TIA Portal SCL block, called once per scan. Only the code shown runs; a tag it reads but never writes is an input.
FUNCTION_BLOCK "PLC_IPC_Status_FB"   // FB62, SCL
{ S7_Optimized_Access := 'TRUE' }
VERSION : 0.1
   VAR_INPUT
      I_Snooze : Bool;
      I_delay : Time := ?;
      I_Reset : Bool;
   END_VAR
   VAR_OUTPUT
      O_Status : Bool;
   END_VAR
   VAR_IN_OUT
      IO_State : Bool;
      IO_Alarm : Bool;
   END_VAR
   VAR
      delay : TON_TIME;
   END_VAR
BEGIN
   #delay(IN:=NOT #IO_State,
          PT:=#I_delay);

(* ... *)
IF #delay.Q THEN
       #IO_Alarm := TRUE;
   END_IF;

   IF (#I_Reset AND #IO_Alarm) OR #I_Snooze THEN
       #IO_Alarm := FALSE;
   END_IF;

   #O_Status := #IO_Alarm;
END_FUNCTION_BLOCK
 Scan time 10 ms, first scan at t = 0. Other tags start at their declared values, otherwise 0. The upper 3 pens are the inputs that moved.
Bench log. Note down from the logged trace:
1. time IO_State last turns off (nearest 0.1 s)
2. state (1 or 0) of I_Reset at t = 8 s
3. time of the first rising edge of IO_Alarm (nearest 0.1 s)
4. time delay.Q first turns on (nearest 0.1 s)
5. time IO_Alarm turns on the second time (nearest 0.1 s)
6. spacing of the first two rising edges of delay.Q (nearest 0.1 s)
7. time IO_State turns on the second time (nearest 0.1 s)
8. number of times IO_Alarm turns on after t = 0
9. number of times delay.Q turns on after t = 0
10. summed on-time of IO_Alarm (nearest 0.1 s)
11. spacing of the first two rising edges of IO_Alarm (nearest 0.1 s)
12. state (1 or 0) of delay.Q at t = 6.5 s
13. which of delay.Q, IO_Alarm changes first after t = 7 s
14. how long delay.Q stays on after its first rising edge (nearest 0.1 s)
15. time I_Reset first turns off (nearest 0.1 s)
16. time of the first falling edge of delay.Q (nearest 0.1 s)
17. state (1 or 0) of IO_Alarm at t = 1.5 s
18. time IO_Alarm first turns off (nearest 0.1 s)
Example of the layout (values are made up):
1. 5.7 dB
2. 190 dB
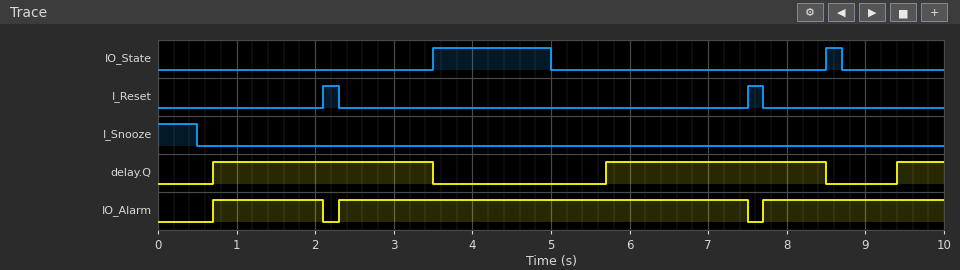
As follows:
1. 8.7 s
2. 0
3. 0.7 s
4. 0.7 s
5. 2.3 s
6. 5.0 s
7. 8.5 s
8. 3
9. 3
10. 8.9 s
11. 1.6 s
12. 1
13. IO_Alarm
14. 2.8 s
15. 2.3 s
16. 3.5 s
17. 1
18. 2.1 s
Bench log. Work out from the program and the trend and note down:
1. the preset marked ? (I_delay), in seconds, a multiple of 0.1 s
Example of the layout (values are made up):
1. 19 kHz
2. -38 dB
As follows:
1. 0.7 s
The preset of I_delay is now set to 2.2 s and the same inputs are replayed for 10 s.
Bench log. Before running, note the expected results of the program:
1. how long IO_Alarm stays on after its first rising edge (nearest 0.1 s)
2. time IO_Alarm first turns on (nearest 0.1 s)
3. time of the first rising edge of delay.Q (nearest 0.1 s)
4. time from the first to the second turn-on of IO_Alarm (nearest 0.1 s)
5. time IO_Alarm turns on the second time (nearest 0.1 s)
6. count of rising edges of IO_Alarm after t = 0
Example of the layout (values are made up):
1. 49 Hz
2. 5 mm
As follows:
1. 5.2 s
2. 2.3 s
3. 2.2 s
4. 5.4 s
5. 7.7 s
6. 2
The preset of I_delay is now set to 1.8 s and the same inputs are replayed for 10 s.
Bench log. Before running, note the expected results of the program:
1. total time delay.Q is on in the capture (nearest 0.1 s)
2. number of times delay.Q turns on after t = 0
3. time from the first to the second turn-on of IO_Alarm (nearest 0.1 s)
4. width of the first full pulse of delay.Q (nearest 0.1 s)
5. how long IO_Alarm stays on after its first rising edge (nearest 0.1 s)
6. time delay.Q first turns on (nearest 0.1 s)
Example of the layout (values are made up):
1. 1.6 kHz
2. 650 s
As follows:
1. 3.4 s
2. 2
3. 0.5 s
4. 1.7 s
5. 0.3 s
6. 1.8 s
